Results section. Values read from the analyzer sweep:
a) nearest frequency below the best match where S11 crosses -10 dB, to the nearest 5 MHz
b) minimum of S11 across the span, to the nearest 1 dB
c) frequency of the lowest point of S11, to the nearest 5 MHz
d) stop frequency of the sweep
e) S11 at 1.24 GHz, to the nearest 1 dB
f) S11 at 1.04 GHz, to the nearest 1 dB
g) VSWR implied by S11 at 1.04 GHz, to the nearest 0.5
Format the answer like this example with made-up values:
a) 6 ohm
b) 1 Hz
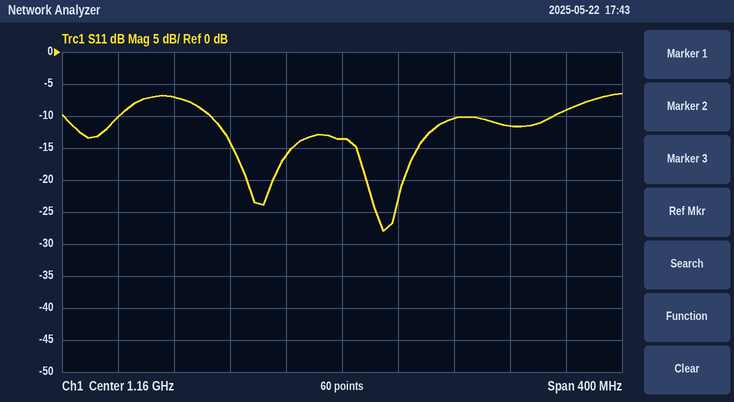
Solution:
a) 1.065 GHz
b) -28 dB
c) 1.190 GHz
d) 1.36 GHz
e) -10 dB
f) -7 dB
g) 2.5
